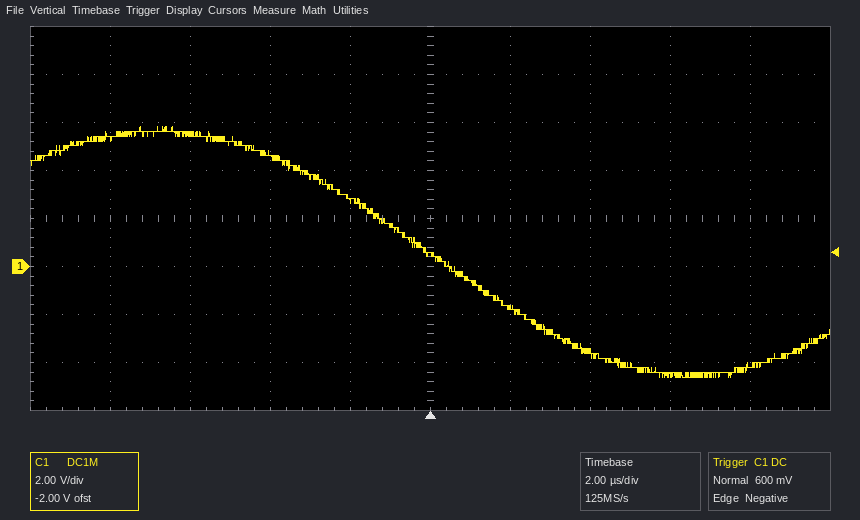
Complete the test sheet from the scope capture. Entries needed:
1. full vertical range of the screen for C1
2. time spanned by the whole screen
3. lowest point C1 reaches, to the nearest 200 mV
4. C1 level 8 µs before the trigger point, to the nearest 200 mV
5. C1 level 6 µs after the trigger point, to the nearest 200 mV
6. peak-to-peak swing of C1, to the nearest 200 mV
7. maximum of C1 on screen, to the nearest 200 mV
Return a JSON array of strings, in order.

["16 V", "20 µs", "-4.6 V", "5.4 V", "-4.6 V", "10.4 V", "5.8 V"]
